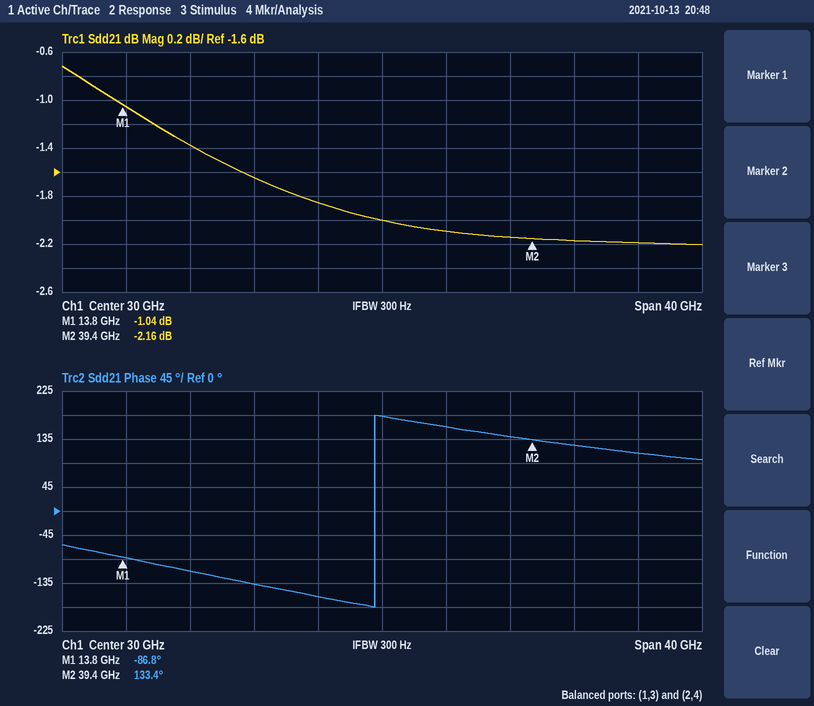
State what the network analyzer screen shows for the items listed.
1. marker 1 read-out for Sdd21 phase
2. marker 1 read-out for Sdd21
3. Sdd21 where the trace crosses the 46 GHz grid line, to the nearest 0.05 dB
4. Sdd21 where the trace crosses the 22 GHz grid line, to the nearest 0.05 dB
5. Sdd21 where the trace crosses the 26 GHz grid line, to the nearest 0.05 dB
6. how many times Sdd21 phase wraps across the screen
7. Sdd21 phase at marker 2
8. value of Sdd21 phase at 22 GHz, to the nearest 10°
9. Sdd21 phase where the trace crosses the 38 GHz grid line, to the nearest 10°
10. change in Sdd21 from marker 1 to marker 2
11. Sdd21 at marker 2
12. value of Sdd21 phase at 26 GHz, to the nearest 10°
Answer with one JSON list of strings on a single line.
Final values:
["-86.8°", "-1.04 dB", "-2.20 dB", "-1.65 dB", "-1.85 dB", "1", "133.4°", "-140°", "140°", "-1.12 dB", "-2.16 dB", "-160°"]
